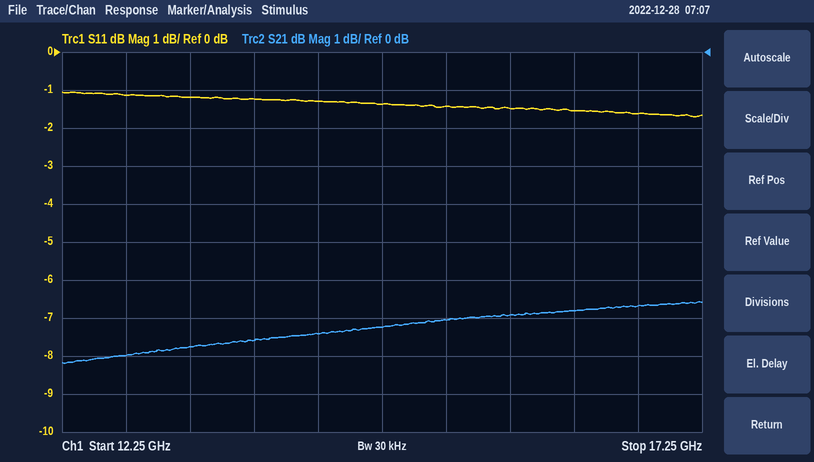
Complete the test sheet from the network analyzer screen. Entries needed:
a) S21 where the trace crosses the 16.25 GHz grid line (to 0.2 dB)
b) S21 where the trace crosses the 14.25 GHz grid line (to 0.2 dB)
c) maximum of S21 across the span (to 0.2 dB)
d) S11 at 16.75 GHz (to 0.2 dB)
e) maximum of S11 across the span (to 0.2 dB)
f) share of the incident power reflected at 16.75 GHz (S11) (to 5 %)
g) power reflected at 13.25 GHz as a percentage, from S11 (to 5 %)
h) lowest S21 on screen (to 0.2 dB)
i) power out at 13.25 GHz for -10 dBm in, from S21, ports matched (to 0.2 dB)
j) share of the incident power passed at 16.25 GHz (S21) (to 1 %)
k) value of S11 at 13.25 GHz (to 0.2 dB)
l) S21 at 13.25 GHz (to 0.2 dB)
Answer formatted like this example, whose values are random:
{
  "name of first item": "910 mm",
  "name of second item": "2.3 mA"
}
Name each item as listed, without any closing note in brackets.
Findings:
{
  "S21 where the trace crosses the 16.25 GHz grid line": "-6.8 dB",
  "S21 where the trace crosses the 14.25 GHz grid line": "-7.4 dB",
  "maximum of S21 across the span": "-6.6 dB",
  "S11 at 16.75 GHz": "-1.6 dB",
  "maximum of S11 across the span": "-1.0 dB",
  "share of the incident power reflected at 16.75 GHz (S11)": "70 %",
  "power reflected at 13.25 GHz as a percentage, from S11": "75 %",
  "lowest S21 on screen": "-8.2 dB",
  "power out at 13.25 GHz for -10 dBm in, from S21, ports matched": "-17.8 dBm",
  "share of the incident power passed at 16.25 GHz (S21)": "21 %",
  "value of S11 at 13.25 GHz": "-1.2 dB",
  "S21 at 13.25 GHz": "-7.8 dB"
}
